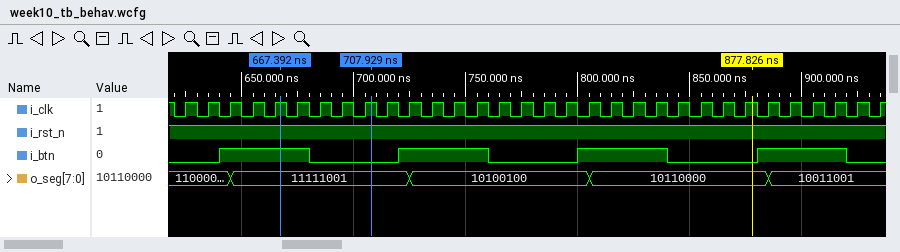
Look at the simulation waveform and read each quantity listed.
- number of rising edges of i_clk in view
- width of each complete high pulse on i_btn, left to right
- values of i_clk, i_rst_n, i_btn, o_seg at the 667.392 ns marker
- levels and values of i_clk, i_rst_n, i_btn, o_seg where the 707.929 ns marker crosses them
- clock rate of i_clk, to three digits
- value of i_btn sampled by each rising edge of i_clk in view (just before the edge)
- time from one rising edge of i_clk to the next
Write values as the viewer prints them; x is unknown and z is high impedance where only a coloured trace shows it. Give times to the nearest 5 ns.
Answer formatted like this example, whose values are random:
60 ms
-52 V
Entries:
32
40 ns, 40 ns, 40 ns, 40 ns
i_clk=1, i_rst_n=1, i_btn=1, o_seg=11111001
i_clk=1, i_rst_n=1, i_btn=0, o_seg=11111001
100 MHz
0 0 1 1 1 1 0 0 0 0 1 1 1 1 0 0 0 0 1 1 1 1 0 0 0 0 1 1 1 1 0 0
10 ns
